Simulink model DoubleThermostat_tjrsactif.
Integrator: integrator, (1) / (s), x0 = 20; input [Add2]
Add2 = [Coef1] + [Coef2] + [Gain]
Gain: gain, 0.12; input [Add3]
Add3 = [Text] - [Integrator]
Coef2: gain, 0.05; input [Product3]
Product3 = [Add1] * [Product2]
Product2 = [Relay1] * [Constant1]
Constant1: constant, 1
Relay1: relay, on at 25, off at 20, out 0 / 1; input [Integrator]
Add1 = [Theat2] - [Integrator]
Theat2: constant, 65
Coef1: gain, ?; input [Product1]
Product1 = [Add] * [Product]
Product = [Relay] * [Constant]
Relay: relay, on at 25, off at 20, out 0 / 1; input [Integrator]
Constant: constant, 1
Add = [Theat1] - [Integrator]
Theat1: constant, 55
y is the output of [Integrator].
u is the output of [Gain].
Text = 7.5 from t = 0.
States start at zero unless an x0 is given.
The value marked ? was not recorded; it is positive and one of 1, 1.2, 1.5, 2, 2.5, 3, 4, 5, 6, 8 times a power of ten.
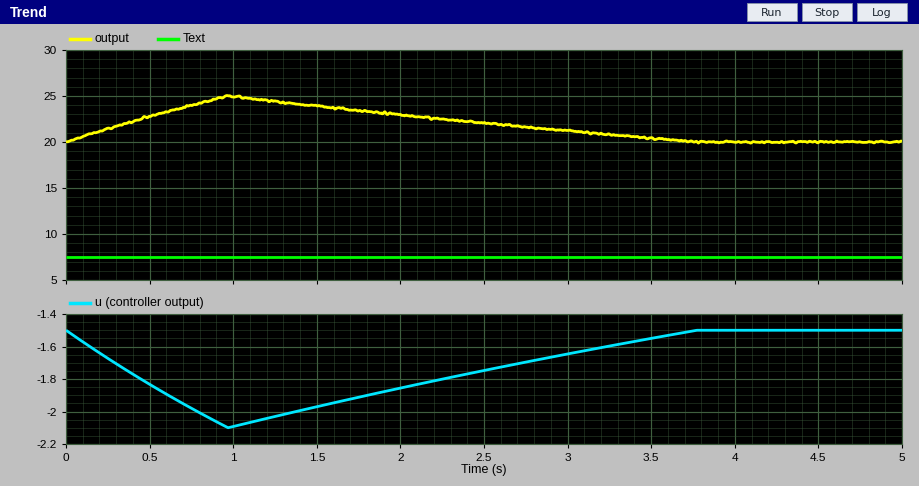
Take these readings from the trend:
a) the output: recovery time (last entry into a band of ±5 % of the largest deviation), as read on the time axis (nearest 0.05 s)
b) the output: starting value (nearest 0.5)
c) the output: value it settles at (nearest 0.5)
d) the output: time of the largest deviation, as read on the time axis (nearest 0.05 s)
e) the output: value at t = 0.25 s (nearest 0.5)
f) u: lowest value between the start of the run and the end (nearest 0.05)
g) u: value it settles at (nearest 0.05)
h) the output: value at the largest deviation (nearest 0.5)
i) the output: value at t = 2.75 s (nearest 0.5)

3.60 s
20.0
20.0
0.95 s
21.5
-2.10
-1.50
25.0
21.5
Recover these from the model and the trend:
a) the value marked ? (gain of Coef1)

0.15
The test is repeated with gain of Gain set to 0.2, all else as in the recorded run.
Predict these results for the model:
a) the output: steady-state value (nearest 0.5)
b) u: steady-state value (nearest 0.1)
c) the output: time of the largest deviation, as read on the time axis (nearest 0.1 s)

20.0
-2.5
1.3 s
